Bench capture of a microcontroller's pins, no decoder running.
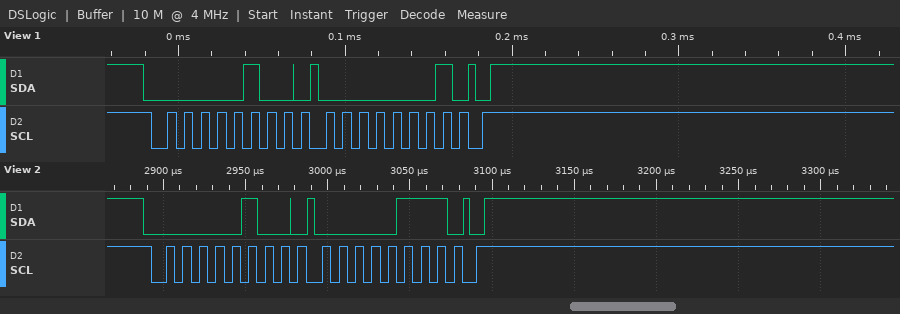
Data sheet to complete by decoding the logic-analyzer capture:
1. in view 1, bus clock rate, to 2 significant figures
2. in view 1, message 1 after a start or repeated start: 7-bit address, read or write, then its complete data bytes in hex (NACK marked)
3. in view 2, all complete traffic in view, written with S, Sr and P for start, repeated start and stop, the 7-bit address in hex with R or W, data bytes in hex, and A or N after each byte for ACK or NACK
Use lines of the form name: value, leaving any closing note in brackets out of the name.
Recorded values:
in view 1, bus clock rate, to 2 significant figures: 100 kHz
in view 1, message 1 after a start or repeated start: 7-bit address, read or write, then its complete data bytes in hex: 0x02 write: 01
in view 2, all complete traffic in view, written with S, Sr and P for start, repeated start and stop, the 7-bit address in hex with R or W, data bytes in hex, and A or N after each byte for ACK or NACK: S 02W A 07 A P
